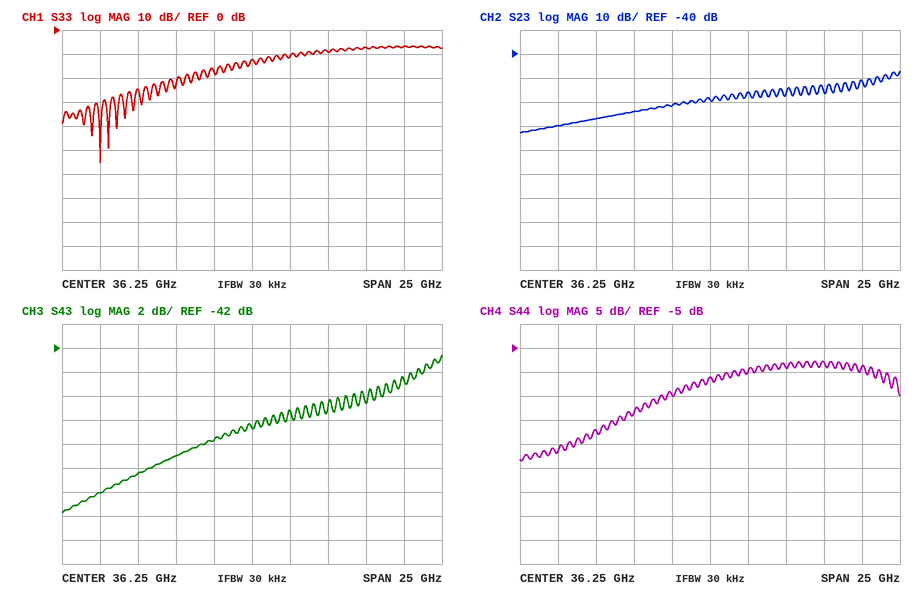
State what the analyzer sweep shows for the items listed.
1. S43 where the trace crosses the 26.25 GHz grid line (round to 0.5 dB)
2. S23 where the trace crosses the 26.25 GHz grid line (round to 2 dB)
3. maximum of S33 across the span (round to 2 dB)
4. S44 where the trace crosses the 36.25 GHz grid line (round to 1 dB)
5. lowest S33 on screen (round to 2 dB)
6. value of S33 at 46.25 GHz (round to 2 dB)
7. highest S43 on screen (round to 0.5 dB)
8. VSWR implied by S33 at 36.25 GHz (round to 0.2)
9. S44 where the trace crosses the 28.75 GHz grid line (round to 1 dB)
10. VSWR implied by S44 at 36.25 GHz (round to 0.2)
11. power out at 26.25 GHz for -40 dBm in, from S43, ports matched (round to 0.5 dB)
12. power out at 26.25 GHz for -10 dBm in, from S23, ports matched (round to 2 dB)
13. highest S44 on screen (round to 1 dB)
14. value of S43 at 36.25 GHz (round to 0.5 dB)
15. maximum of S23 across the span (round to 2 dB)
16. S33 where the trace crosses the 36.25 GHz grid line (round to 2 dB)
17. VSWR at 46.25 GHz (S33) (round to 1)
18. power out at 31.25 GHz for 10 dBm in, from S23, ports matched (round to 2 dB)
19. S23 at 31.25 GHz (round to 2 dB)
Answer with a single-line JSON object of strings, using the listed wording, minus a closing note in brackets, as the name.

{"S43 where the trace crosses the 26.25 GHz grid line": "-54.0 dB", "S23 where the trace crosses the 26.25 GHz grid line": "-70 dB", "maximum of S33 across the span": "-6 dB", "S44 where the trace crosses the 36.25 GHz grid line": "-11 dB", "lowest S33 on screen": "-56 dB", "value of S33 at 46.25 GHz": "-6 dB", "highest S43 on screen": "-42.5 dB", "VSWR implied by S33 at 36.25 GHz": "1.6", "S44 where the trace crosses the 28.75 GHz grid line": "-22 dB", "VSWR implied by S44 at 36.25 GHz": "1.8", "power out at 26.25 GHz for -40 dBm in, from S43, ports matched": "-94.0 dBm", "power out at 26.25 GHz for -10 dBm in, from S23, ports matched": "-80 dBm", "highest S44 on screen": "-8 dB", "value of S43 at 36.25 GHz": "-48.5 dB", "maximum of S23 across the span": "-48 dB", "S33 where the trace crosses the 36.25 GHz grid line": "-12 dB", "VSWR at 46.25 GHz (S33)": "3", "power out at 31.25 GHz for 10 dBm in, from S23, ports matched": "-54 dBm", "S23 at 31.25 GHz": "-64 dB"}
